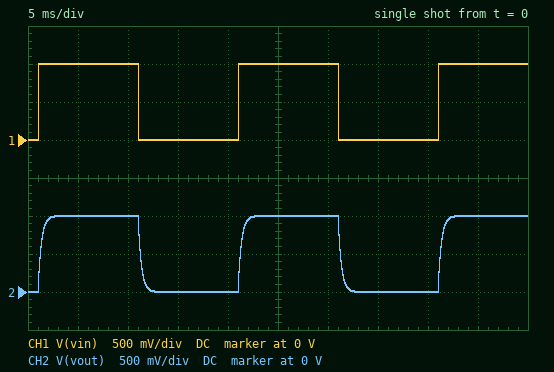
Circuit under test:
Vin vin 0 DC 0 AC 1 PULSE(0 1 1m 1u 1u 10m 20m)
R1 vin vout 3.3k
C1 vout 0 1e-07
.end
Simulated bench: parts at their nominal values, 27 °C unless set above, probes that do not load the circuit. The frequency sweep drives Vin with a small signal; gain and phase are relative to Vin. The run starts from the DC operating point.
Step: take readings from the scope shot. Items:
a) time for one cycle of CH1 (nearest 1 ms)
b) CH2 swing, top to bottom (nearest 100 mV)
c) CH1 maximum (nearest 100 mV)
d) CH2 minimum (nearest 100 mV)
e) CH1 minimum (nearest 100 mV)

20 ms
1.0 V
1.0 V
0 V
0 V
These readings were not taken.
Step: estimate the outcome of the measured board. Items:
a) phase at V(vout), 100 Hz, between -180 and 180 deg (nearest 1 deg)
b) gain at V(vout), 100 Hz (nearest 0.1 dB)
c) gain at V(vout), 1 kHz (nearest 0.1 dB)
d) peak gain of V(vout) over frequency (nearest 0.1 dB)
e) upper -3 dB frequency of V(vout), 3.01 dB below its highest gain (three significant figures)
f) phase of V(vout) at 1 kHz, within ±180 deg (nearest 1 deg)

-12 deg
-0.2 dB
-7.2 dB
0 dB
482 Hz
-64 deg
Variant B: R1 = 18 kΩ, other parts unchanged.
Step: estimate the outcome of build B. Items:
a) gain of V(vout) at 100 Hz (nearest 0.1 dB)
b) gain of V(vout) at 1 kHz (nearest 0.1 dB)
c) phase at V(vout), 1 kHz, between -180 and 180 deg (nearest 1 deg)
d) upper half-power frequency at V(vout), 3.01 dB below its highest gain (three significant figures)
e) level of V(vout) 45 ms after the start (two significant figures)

-3.6 dB
-21.1 dB
-85 deg
88.4 Hz
890 mV
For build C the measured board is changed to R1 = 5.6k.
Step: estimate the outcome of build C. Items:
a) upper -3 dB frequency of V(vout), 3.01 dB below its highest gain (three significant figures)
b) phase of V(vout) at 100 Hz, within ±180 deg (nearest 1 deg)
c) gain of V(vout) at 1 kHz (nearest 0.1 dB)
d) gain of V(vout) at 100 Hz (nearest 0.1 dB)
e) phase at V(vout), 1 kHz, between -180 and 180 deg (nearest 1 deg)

284 Hz
-19 deg
-11.3 dB
-0.5 dB
-74 deg
